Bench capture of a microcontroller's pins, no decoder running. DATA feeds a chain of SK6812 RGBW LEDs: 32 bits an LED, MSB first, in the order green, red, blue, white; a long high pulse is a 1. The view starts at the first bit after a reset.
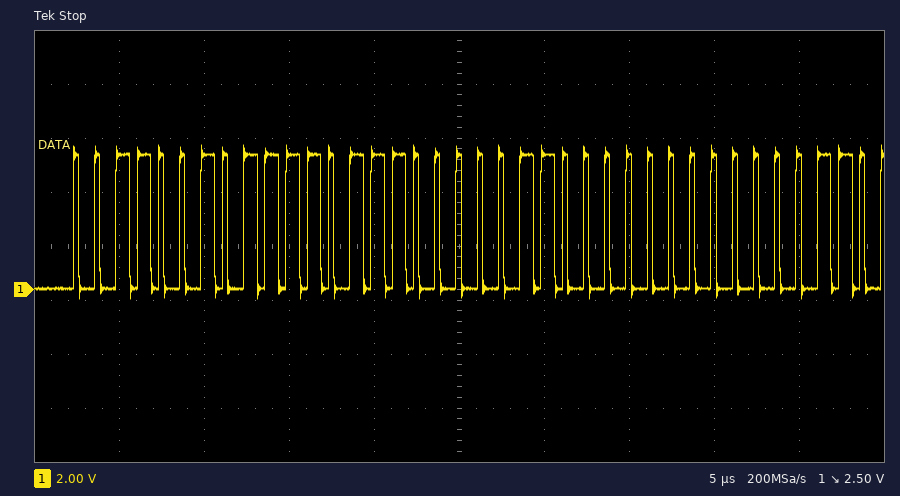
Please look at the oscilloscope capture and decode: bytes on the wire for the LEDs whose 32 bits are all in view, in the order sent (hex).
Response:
32 F7 06 00
